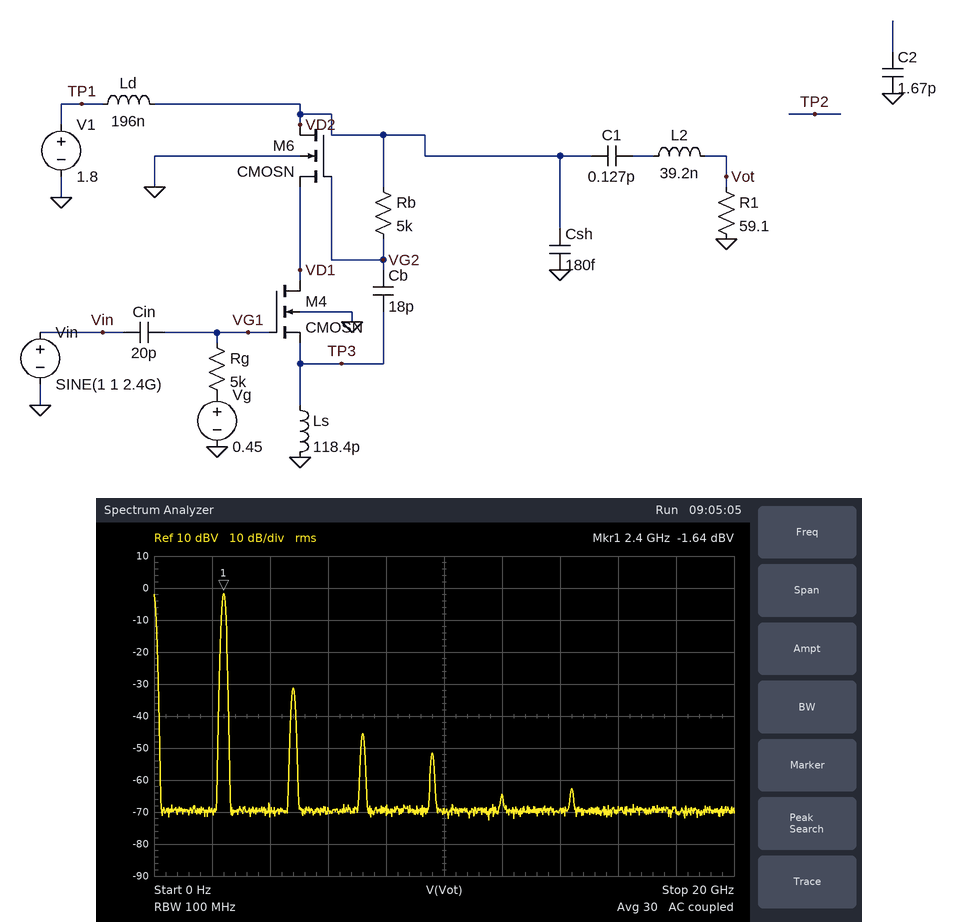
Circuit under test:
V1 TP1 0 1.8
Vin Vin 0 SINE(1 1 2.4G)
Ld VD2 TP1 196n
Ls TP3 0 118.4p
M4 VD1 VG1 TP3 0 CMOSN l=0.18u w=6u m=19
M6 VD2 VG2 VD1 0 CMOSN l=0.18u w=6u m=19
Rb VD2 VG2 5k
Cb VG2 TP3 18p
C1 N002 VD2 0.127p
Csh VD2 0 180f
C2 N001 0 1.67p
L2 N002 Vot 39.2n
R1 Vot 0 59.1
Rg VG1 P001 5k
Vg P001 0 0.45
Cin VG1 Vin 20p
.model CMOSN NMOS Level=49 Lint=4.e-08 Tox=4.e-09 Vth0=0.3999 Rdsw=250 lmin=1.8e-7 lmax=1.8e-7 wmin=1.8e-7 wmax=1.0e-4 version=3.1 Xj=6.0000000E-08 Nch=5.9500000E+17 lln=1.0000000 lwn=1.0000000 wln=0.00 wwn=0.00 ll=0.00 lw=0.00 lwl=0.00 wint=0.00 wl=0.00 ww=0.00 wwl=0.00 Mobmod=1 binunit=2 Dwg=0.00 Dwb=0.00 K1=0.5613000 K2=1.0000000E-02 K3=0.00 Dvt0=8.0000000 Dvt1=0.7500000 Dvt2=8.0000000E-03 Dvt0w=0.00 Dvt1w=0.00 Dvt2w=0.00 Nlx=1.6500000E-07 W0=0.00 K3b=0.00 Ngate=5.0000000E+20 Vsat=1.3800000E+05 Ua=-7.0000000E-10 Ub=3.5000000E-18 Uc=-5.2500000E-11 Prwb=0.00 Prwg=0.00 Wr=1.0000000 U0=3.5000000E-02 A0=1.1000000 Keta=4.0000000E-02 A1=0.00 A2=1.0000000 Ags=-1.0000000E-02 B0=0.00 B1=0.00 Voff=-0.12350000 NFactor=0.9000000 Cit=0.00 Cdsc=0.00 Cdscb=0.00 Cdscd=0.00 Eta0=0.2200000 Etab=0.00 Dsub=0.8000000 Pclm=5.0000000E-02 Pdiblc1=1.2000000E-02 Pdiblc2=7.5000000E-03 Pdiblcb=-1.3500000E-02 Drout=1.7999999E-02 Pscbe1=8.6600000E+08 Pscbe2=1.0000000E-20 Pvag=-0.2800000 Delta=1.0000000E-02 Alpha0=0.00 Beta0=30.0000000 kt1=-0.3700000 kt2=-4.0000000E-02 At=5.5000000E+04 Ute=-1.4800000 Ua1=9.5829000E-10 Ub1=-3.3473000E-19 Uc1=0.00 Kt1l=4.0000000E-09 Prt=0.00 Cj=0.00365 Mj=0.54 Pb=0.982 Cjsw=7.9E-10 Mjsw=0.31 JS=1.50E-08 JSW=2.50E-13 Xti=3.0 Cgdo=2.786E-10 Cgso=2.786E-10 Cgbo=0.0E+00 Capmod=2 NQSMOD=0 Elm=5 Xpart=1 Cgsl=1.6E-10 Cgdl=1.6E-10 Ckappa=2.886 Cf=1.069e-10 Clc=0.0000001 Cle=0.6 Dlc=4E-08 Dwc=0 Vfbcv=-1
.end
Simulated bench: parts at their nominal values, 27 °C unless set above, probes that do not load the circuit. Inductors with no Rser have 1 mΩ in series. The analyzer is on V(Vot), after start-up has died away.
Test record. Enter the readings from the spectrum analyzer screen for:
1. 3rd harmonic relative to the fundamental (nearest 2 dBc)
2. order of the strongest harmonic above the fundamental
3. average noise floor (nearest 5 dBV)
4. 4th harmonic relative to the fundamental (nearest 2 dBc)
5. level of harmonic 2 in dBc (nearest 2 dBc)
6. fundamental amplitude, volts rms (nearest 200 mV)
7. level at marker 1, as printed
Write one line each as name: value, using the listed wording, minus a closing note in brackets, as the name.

3rd harmonic relative to the fundamental: -44 dBc
order of the strongest harmonic above the fundamental: 2
average noise floor: -70 dBV
4th harmonic relative to the fundamental: -50 dBc
level of harmonic 2 in dBc: -30 dBc
fundamental amplitude, volts rms: 800 mV
level at marker 1, as printed: -1.64 dBV
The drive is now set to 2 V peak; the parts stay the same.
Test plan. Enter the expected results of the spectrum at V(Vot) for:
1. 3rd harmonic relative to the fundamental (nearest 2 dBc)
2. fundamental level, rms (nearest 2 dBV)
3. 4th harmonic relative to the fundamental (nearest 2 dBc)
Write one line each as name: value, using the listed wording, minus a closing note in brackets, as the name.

3rd harmonic relative to the fundamental: -42 dBc
fundamental level, rms: 0 dBV
4th harmonic relative to the fundamental: -56 dBc
